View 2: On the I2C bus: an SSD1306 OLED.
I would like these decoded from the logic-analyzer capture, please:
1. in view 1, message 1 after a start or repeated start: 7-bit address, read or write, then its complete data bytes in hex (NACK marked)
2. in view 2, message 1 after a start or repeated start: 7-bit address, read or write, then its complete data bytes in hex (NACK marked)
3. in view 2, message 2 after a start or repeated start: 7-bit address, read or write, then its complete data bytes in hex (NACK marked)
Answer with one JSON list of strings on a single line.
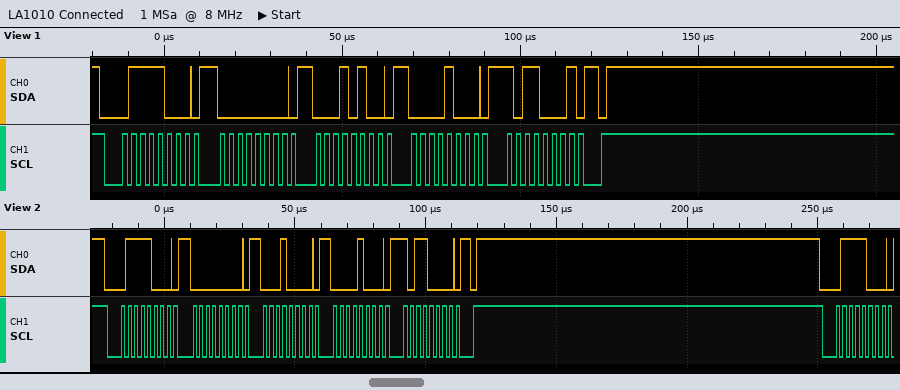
["0x3C write: 00 14 08 B1", "0x3C write: 00 10 08 B0", "0x3C write"]
